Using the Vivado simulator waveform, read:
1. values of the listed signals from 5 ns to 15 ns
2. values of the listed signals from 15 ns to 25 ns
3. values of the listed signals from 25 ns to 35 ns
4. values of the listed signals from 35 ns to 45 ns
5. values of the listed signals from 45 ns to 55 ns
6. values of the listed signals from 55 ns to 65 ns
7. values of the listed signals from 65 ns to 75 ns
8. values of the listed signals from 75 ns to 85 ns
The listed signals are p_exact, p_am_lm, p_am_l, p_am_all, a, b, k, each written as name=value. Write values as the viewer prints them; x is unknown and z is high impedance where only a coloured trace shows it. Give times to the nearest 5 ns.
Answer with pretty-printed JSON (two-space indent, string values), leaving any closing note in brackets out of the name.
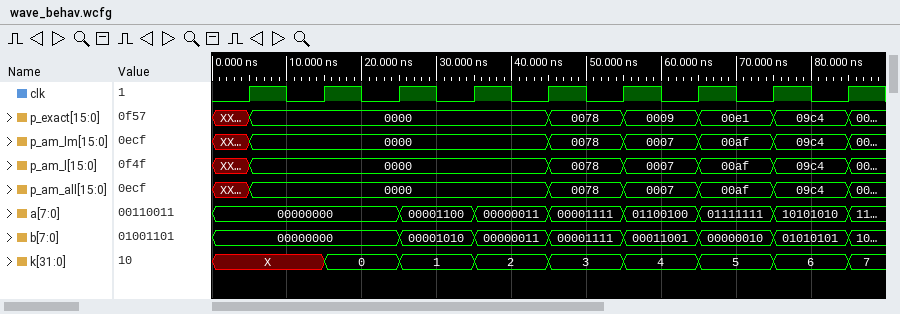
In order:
{
  "values of the listed signals from 5 ns to 15 ns": "p_exact=0000, p_am_lm=0000, p_am_l=0000, p_am_all=0000, a=00000000, b=00000000, k=X",
  "values of the listed signals from 15 ns to 25 ns": "p_exact=0000, p_am_lm=0000, p_am_l=0000, p_am_all=0000, a=00000000, b=00000000, k=0",
  "values of the listed signals from 25 ns to 35 ns": "p_exact=0000, p_am_lm=0000, p_am_l=0000, p_am_all=0000, a=00001100, b=00001010, k=1",
  "values of the listed signals from 35 ns to 45 ns": "p_exact=0000, p_am_lm=0000, p_am_l=0000, p_am_all=0000, a=00000011, b=00000011, k=2",
  "values of the listed signals from 45 ns to 55 ns": "p_exact=0078, p_am_lm=0078, p_am_l=0078, p_am_all=0078, a=00001111, b=00001111, k=3",
  "values of the listed signals from 55 ns to 65 ns": "p_exact=0009, p_am_lm=0007, p_am_l=0007, p_am_all=0007, a=01100100, b=00011001, k=4",
  "values of the listed signals from 65 ns to 75 ns": "p_exact=00e1, p_am_lm=00af, p_am_l=00af, p_am_all=00af, a=01111111, b=00000010, k=5",
  "values of the listed signals from 75 ns to 85 ns": "p_exact=09c4, p_am_lm=09c4, p_am_l=09c4, p_am_all=09c4, a=10101010, b=01010101, k=6"
}
